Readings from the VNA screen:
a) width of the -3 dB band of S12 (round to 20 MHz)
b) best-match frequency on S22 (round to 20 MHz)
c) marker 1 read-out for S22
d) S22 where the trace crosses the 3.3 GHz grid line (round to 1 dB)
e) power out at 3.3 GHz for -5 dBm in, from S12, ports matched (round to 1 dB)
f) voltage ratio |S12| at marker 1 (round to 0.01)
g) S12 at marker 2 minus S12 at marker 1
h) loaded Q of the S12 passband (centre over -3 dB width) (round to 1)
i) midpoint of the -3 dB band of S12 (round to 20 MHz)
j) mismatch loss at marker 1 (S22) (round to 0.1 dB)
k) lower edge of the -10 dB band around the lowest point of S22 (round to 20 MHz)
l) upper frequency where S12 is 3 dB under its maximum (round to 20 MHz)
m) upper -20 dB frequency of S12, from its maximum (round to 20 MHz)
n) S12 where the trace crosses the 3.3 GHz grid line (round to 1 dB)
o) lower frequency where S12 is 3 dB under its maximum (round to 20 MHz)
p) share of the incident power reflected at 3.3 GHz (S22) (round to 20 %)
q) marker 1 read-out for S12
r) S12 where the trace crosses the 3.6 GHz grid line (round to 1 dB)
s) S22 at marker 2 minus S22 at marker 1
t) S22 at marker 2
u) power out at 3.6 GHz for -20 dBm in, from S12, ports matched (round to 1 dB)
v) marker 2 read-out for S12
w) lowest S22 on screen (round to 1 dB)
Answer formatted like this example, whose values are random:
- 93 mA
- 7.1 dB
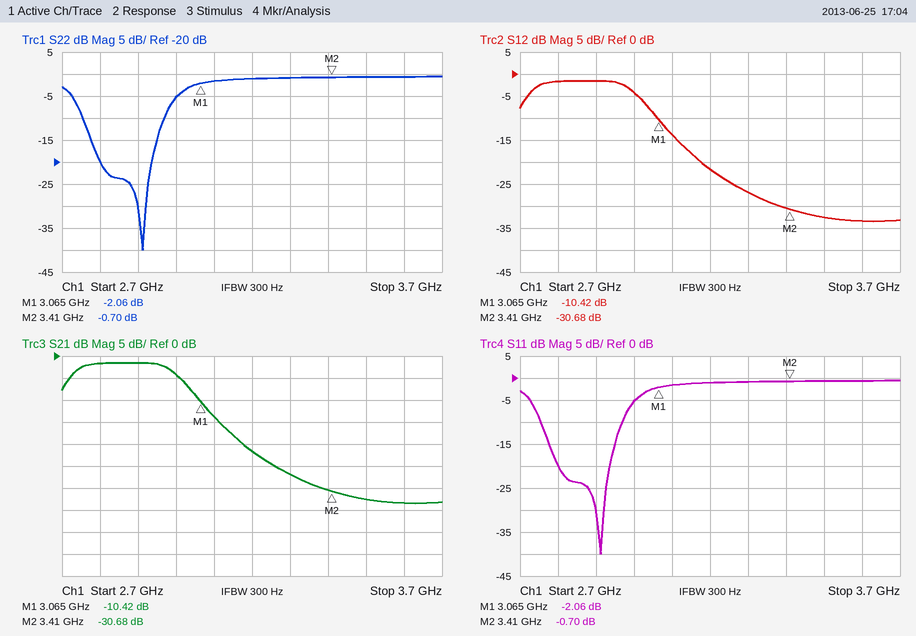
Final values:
- 280 MHz
- 2.92 GHz
- -2.06 dB
- -1 dB
- -32 dBm
- 0.30
- -20.26 dB
- 10
- 2.86 GHz
- 4.2 dB
- 2.76 GHz
- 3.00 GHz
- 3.20 GHz
- -27 dB
- 2.72 GHz
- 80 %
- -10.42 dB
- -33 dB
- 1.36 dB
- -0.70 dB
- -53 dBm
- -30.68 dB
- -40 dB
